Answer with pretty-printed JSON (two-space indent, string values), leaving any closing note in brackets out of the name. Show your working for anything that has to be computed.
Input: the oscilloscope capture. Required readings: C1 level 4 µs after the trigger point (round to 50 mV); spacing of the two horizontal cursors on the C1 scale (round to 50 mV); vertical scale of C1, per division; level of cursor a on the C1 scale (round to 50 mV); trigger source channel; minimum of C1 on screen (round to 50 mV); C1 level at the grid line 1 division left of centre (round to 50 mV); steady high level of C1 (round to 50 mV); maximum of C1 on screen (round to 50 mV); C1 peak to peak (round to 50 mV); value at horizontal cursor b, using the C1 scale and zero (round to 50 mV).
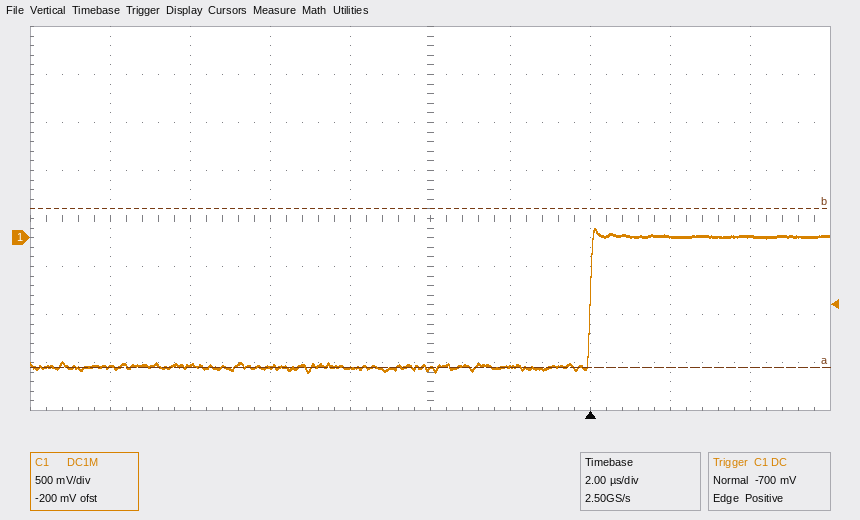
{
  "C1 level 4 µs after the trigger point": "0 mV",
  "spacing of the two horizontal cursors on the C1 scale": "1.65 V",
  "vertical scale of C1, per division": "500 mV",
  "level of cursor a on the C1 scale": "-1.35 V",
  "trigger source channel": "C1",
  "minimum of C1 on screen": "-1.40 V",
  "C1 level at the grid line 1 division left of centre": "-1.35 V",
  "steady high level of C1": "0 mV",
  "maximum of C1 on screen": "100 mV",
  "C1 peak to peak": "100 mV − (-1.40 V) = 1.50 V",
  "value at horizontal cursor b, using the C1 scale and zero": "300 mV"
}
